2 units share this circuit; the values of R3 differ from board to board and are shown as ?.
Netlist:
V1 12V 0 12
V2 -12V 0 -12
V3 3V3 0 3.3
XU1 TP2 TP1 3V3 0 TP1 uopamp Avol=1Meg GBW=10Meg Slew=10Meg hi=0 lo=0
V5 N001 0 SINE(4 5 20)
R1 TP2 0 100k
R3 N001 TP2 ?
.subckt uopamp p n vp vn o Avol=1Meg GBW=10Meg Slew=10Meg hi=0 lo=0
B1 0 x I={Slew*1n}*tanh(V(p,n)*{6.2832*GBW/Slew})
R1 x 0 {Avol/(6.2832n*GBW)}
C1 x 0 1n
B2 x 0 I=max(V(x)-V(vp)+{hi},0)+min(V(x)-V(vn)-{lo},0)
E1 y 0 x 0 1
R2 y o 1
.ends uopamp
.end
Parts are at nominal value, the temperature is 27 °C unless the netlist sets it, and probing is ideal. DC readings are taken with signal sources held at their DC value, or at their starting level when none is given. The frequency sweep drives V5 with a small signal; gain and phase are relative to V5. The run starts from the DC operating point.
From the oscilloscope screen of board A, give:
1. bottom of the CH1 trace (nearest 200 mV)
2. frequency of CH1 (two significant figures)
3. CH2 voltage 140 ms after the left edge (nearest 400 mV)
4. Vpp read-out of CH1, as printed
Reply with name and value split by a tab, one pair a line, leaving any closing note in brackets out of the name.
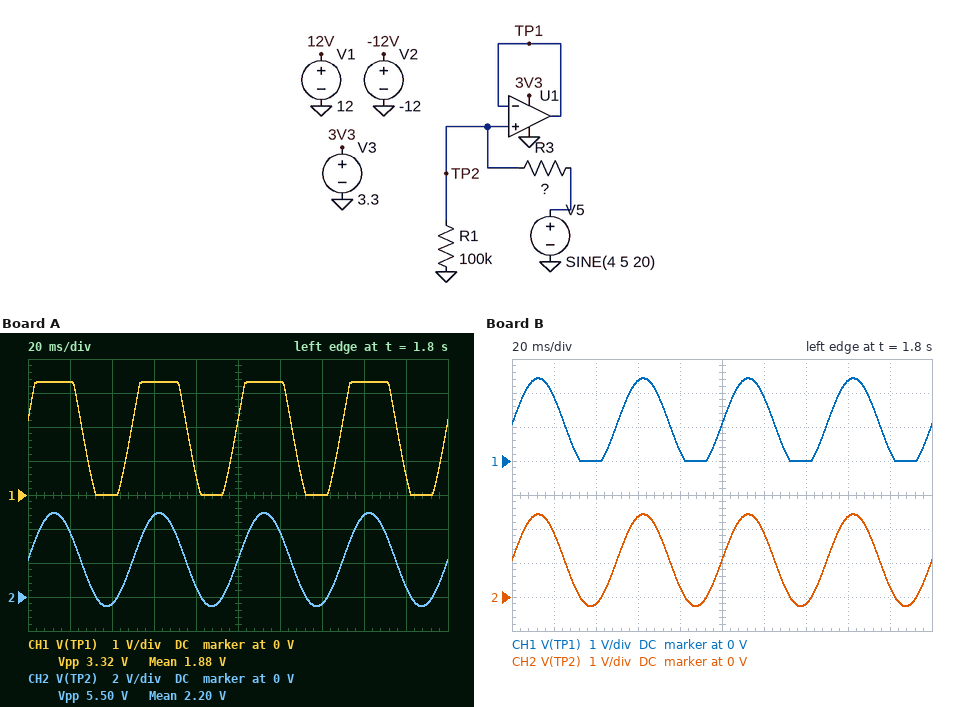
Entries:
bottom of the CH1 trace	0 V
frequency of CH1	20 Hz
CH2 voltage 140 ms after the left edge	-400 mV
Vpp read-out of CH1, as printed	3.32 V
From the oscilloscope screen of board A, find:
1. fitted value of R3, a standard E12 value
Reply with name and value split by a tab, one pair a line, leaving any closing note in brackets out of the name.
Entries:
fitted value of R3, a standard E12 value	82 kΩ
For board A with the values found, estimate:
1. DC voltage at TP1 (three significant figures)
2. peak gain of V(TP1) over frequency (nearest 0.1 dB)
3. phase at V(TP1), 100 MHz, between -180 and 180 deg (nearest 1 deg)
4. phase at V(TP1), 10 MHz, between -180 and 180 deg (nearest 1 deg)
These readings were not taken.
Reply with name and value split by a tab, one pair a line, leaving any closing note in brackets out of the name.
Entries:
DC voltage at TP1	2.20 V
peak gain of V(TP1) over frequency	-5.2 dB
phase at V(TP1), 100 MHz, between -180 and 180 deg	-84 deg
phase at V(TP1), 10 MHz, between -180 and 180 deg	-45 deg
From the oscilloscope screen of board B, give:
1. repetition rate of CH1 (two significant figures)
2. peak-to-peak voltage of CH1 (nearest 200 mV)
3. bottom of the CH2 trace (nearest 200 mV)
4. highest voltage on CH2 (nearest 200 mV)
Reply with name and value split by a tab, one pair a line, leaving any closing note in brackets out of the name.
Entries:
repetition rate of CH1	20 Hz
peak-to-peak voltage of CH1	2.4 V
bottom of the CH2 trace	-200 mV
highest voltage on CH2	2.4 V
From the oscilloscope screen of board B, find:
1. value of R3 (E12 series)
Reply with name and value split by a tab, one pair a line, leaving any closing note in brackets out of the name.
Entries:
value of R3	270 kΩ
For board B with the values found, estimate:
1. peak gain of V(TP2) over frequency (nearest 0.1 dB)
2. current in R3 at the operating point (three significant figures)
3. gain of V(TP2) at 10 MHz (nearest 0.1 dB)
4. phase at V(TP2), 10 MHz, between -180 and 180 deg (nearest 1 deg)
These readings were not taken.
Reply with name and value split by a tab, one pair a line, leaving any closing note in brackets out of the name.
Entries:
peak gain of V(TP2) over frequency	-11.4 dB
current in R3 at the operating point	10.8 µA
gain of V(TP2) at 10 MHz	-11.4 dB
phase at V(TP2), 10 MHz, between -180 and 180 deg	0 deg
